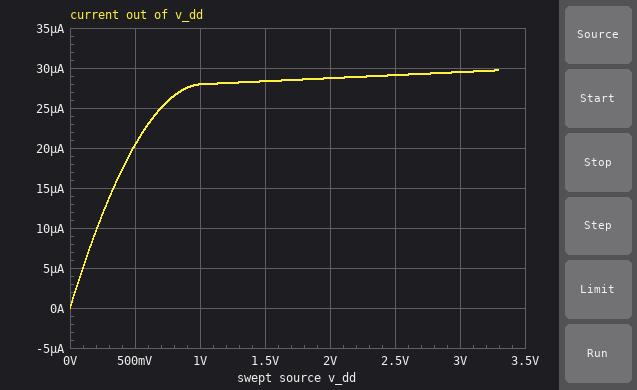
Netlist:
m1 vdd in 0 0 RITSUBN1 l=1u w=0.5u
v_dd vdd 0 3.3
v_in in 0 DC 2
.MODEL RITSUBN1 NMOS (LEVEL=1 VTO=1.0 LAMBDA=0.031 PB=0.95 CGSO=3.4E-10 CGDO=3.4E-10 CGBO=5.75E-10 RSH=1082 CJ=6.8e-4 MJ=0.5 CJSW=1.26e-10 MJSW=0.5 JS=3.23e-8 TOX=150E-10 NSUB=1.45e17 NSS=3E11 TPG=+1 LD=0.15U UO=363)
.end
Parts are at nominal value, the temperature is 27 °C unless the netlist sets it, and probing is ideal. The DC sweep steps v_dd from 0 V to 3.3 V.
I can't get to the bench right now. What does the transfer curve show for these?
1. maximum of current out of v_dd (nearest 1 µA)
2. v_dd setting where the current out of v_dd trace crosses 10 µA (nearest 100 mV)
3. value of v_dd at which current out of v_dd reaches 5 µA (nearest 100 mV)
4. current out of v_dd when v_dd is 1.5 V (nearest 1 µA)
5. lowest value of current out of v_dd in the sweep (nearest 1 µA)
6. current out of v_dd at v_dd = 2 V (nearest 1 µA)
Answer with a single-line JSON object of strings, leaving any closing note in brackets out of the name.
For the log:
{"maximum of current out of v_dd": "30 µA", "v_dd setting where the current out of v_dd trace crosses 10 µA": "200 mV", "value of v_dd at which current out of v_dd reaches 5 µA": "100 mV", "current out of v_dd when v_dd is 1.5 V": "28 µA", "lowest value of current out of v_dd in the sweep": "0 A", "current out of v_dd at v_dd = 2 V": "29 µA"}
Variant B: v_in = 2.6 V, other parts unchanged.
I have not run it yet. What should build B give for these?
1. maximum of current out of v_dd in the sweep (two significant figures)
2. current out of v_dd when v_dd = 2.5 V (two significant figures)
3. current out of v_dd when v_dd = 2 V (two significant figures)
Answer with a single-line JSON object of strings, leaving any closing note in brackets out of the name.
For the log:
{"maximum of current out of v_dd in the sweep": "72 µA", "current out of v_dd when v_dd = 2.5 V": "71 µA", "current out of v_dd when v_dd = 2 V": "70 µA"}
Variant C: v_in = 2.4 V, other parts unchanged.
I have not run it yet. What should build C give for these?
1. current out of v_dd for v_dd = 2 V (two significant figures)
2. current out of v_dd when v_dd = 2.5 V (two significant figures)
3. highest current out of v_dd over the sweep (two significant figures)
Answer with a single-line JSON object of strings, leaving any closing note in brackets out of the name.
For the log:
{"current out of v_dd for v_dd = 2 V": "54 µA", "current out of v_dd when v_dd = 2.5 V": "55 µA", "highest current out of v_dd over the sweep": "56 µA"}
